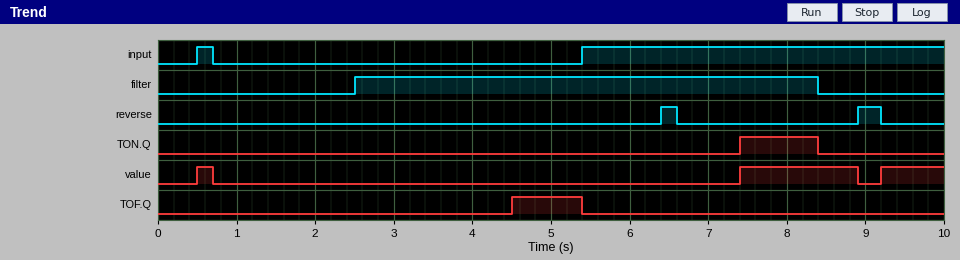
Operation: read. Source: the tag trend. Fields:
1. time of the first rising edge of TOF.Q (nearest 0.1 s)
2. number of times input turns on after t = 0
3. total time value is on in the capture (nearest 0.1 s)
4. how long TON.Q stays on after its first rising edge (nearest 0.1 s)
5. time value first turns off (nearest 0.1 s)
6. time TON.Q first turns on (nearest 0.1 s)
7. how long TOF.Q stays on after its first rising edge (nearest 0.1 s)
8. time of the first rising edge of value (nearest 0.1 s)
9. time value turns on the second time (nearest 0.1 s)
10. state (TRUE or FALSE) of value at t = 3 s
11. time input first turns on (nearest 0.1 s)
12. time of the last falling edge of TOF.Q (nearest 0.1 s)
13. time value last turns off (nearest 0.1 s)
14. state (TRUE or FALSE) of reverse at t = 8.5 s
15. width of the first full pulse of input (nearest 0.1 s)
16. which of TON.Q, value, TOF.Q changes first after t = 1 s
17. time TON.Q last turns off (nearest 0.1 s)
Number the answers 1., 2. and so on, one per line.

1. 4.5 s
2. 2
3. 2.5 s
4. 1.0 s
5. 0.7 s
6. 7.4 s
7. 0.9 s
8. 0.5 s
9. 7.4 s
10. FALSE
11. 0.5 s
12. 5.4 s
13. 8.9 s
14. FALSE
15. 0.2 s
16. TOF.Q
17. 8.4 s
